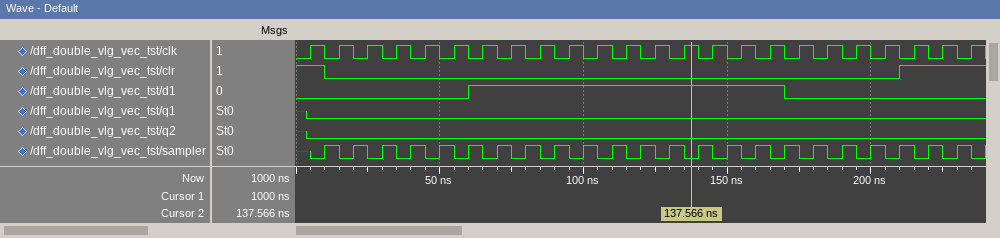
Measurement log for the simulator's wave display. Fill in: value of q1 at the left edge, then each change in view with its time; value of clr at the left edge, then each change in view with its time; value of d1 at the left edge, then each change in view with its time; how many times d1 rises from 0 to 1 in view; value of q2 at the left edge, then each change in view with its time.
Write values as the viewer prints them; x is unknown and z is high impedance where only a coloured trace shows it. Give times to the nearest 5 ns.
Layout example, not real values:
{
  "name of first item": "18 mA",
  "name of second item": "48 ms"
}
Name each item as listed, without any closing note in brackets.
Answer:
{
  "value of q1 at the left edge, then each change in view with its time": "x, 0 at 5 ns",
  "value of clr at the left edge, then each change in view with its time": "1, 0 at 10 ns, 1 at 210 ns",
  "value of d1 at the left edge, then each change in view with its time": "0, 1 at 60 ns, 0 at 170 ns",
  "how many times d1 rises from 0 to 1 in view": "1",
  "value of q2 at the left edge, then each change in view with its time": "x, 0 at 5 ns"
}
